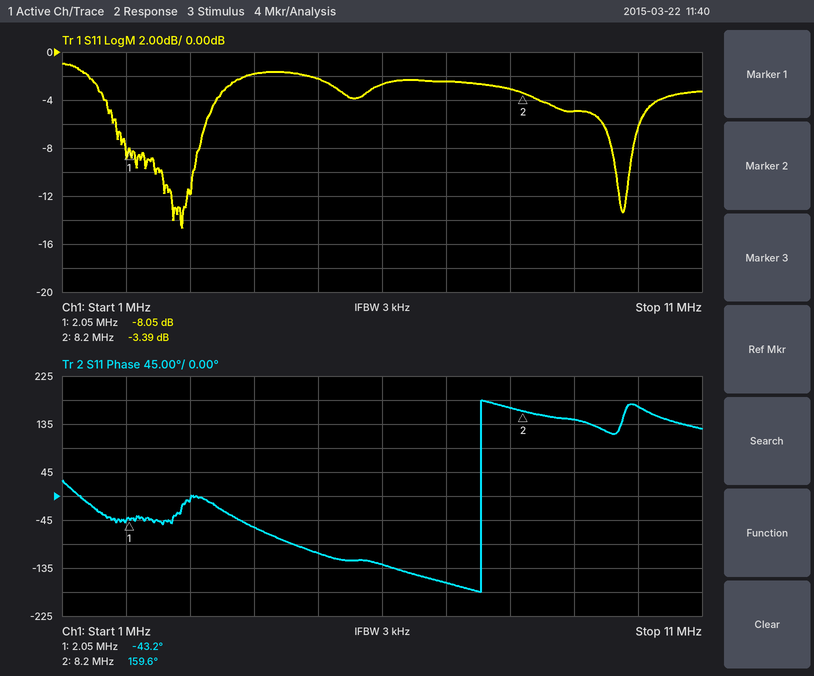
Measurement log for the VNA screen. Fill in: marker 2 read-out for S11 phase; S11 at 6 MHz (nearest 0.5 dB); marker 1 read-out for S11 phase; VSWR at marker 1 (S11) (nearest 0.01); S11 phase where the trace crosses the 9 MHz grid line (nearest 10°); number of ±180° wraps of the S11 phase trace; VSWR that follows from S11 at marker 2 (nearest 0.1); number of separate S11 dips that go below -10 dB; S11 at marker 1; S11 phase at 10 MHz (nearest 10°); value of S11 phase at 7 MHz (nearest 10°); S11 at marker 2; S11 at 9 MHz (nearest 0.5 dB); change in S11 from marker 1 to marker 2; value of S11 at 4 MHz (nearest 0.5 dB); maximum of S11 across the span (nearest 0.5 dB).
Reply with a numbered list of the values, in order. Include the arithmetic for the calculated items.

1. 159.6°
2. -2.5 dB
3. -43.2°
4. (1 + 0.3958)/(1 − 0.3958) ≈ 2.31
5. 140°
6. 1
7. (1 + 0.6769)/(1 − 0.6769) ≈ 5.2
8. 2
9. -8.05 dB
10. 170°
11. -160°
12. -3.39 dB
13. -5.0 dB
14. -3.39 − (-8.05) = 4.66 dB
15. -2.0 dB
16. -1.0 dB
